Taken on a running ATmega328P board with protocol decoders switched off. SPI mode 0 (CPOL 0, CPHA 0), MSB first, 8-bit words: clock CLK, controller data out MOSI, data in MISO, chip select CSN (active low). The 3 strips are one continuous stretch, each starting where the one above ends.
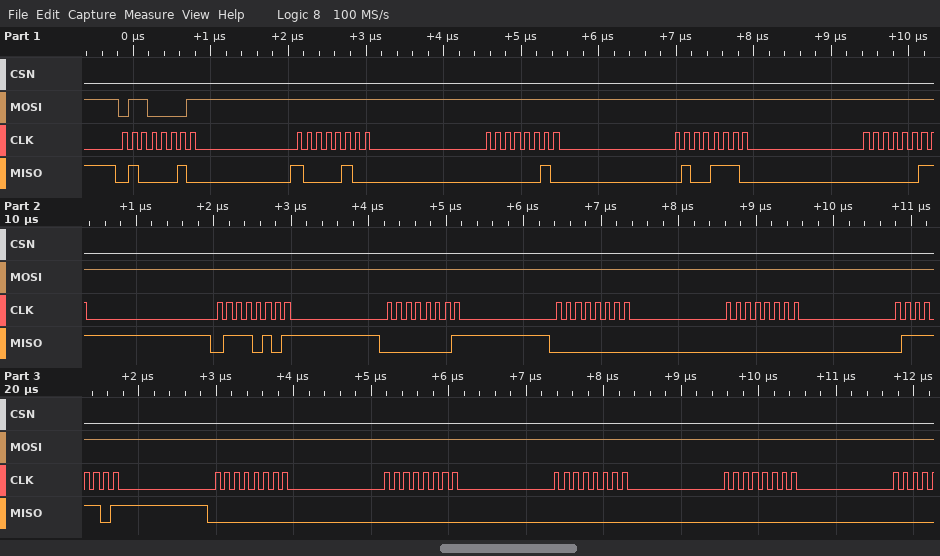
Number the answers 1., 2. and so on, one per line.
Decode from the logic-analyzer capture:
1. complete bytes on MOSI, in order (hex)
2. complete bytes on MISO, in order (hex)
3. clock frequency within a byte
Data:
1. 61 FF FF FF FF FF FF FF FF FF FF FF FF FF
2. 42 84 02 4E 03 75 01 00 00 7D 00 00 00 00
3. 8 MHz
